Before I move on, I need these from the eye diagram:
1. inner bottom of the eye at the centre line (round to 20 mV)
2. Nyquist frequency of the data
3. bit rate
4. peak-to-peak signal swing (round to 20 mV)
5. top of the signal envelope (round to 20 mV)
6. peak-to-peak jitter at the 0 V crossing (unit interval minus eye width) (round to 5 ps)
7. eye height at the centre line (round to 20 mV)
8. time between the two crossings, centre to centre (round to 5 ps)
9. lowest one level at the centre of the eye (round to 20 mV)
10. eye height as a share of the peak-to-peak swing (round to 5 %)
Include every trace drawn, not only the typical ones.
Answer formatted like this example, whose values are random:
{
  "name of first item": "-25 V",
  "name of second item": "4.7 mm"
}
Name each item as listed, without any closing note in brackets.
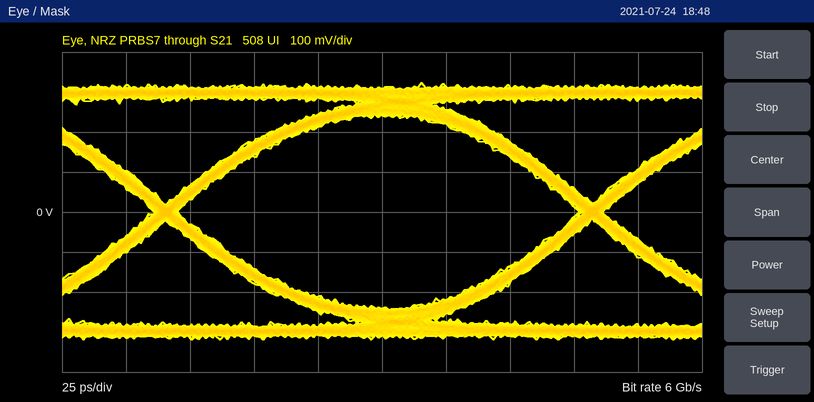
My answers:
{
  "inner bottom of the eye at the centre line": "-240 mV",
  "Nyquist frequency of the data": "3 GHz",
  "bit rate": "6 Gb/s",
  "peak-to-peak signal swing": "640 mV",
  "top of the signal envelope": "320 mV",
  "peak-to-peak jitter at the 0 V crossing (unit interval minus eye width)": "10 ps",
  "eye height at the centre line": "480 mV",
  "time between the two crossings, centre to centre": "165 ps",
  "lowest one level at the centre of the eye": "240 mV",
  "eye height as a share of the peak-to-peak swing": "75 %"
}
